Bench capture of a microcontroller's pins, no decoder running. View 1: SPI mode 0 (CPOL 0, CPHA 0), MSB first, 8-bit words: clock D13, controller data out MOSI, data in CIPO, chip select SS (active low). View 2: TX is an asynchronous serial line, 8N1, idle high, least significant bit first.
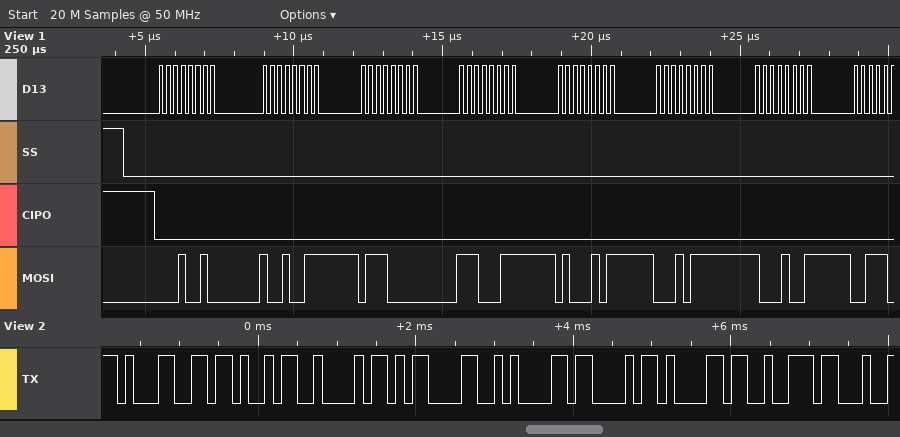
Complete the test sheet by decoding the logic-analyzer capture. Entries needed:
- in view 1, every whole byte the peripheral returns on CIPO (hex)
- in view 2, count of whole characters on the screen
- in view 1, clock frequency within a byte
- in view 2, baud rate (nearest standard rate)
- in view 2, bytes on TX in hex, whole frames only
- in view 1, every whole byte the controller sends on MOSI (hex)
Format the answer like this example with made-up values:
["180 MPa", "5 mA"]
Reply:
["00 00 00 00 00 00 00", "8", "4 MHz", "9600 baud", "31 4B 42 0D 0A 43 61 72", "12 93 70 E3 45 17 89"]
